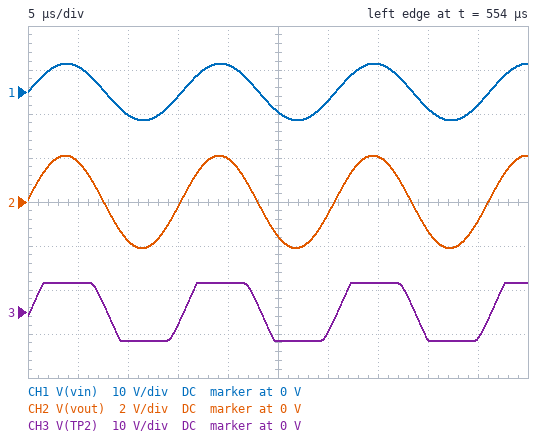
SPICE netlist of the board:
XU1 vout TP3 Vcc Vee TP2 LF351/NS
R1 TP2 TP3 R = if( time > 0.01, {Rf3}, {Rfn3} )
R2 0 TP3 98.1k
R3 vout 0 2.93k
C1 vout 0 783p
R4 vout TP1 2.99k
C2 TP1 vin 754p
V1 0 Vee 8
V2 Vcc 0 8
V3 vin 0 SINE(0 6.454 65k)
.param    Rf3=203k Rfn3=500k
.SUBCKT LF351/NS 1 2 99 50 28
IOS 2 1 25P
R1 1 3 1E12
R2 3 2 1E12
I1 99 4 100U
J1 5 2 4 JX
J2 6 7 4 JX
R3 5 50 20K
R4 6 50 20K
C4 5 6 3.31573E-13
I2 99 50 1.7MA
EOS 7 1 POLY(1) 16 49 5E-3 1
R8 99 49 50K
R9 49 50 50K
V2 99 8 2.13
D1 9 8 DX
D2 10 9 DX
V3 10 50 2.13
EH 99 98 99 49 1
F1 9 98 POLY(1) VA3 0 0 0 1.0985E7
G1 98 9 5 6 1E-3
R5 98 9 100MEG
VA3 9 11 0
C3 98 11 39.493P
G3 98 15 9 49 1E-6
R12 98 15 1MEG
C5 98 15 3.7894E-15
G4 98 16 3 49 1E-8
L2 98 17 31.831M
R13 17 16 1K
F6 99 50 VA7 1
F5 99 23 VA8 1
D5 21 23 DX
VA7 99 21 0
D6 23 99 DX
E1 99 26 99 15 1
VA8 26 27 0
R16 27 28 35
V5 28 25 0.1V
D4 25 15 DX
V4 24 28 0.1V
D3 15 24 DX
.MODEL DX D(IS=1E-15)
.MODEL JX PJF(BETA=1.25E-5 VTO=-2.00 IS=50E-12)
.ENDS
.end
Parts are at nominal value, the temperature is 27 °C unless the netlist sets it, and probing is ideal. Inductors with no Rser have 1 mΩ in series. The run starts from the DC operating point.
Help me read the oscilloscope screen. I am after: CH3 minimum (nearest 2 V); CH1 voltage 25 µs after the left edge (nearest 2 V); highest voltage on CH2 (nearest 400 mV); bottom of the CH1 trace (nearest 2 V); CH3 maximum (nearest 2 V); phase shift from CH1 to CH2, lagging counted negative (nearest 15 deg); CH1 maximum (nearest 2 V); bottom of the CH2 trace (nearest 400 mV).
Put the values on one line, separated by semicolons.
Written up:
-6 V; -4 V; 2.0 V; -6 V; 6 V; 0 deg; 6 V; -2.0 V
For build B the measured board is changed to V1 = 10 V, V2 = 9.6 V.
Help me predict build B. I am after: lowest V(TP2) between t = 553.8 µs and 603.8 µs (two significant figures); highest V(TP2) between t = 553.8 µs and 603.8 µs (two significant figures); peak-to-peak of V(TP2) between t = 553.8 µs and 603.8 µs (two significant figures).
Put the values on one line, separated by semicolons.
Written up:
-8.6 V; 8.2 V; 17 V
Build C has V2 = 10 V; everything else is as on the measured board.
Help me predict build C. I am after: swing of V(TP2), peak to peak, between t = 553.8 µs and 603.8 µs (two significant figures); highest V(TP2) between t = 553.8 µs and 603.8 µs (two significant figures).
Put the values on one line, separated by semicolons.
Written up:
15 V; 8.6 V
